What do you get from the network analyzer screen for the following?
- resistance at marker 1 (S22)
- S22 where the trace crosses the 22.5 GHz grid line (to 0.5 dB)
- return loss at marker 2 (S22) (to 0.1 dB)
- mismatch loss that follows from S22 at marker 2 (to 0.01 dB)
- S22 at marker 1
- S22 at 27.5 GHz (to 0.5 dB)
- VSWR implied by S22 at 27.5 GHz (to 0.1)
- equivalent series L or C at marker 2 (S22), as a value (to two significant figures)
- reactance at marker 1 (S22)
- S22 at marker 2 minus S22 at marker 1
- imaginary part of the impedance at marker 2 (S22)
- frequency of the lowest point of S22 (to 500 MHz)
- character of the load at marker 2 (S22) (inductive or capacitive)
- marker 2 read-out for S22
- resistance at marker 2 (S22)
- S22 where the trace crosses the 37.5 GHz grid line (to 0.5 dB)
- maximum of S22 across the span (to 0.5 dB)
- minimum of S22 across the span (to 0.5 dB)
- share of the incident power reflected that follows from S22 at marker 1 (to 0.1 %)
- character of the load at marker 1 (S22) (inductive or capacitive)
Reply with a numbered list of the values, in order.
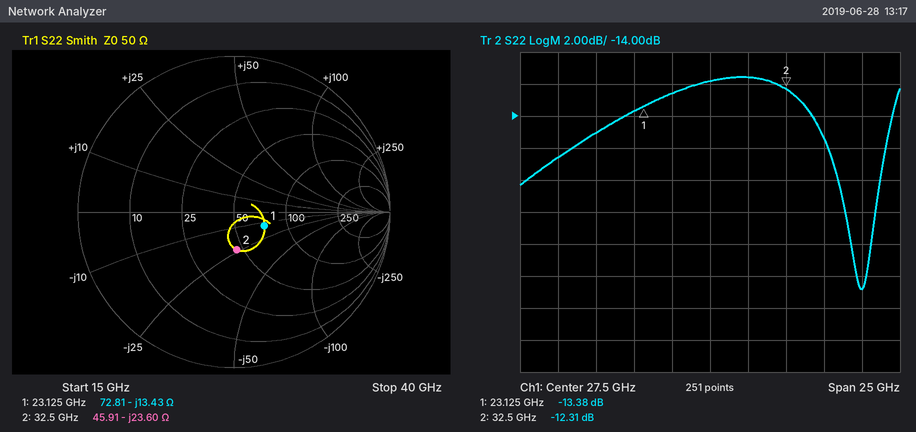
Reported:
1. 72.81 Ω
2. -13.5 dB
3. 12.3 dB
4. 0.26 dB
5. -13.38 dB
6. -12.0 dB
7. 1.7
8. 210 fF
9. -13.43 Ω
10. 1.07 dB
11. -23.60 Ω
12. 37.5 GHz
13. capacitive
14. -12.31 dB
15. 45.91 Ω
16. -25.0 dB
17. -11.5 dB
18. -25.0 dB
19. 4.6 %
20. capacitive
